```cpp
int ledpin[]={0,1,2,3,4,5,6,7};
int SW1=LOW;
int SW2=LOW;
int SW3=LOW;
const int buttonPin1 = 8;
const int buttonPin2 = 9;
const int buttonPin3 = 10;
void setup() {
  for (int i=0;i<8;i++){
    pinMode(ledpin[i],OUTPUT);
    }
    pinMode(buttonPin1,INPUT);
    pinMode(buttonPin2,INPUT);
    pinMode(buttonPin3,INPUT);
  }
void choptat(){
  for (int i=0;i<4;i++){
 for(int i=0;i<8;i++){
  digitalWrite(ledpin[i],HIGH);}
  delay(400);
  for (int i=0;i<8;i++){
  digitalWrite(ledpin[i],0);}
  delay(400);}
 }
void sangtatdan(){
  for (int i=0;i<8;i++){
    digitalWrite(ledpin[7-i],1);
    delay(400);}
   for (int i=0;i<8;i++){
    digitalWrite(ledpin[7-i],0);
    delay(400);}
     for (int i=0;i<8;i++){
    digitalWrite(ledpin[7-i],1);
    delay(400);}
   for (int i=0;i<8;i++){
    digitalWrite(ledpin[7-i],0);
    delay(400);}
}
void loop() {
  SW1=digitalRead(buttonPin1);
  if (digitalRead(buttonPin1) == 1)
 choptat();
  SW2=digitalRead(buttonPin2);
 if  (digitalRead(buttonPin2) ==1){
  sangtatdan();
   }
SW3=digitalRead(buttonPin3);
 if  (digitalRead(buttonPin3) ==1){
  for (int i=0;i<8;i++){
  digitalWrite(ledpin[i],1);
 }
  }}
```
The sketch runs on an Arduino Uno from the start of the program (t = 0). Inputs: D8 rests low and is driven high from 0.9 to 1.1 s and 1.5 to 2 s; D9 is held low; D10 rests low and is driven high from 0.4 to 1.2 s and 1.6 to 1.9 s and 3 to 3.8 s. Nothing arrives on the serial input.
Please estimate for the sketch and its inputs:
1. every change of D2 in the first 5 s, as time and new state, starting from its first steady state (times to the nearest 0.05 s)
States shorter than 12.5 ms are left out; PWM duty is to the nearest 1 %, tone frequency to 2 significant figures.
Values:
0 s low; 0.4 s high; 1.3 s low; 1.7 s high; 2.1 s low; 2.5 s high; 2.9 s low; 3.3 s high; 3.7 s low
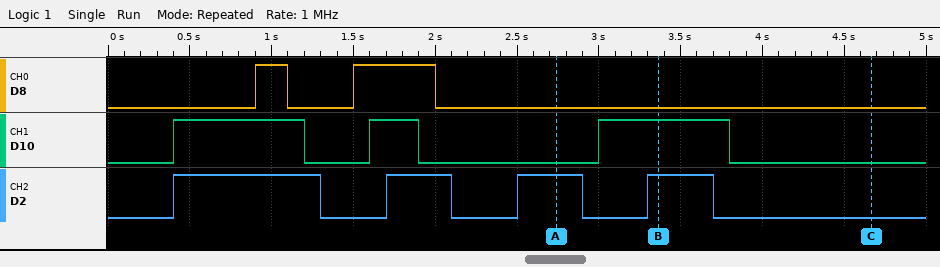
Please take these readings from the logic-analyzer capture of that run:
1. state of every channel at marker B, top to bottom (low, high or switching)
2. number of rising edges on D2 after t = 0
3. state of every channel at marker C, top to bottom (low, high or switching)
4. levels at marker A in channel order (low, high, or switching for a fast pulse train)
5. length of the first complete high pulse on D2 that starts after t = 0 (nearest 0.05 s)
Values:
D8 low, D10 high, D2 high
4
D8 low, D10 low, D2 low
D8 low, D10 low, D2 high
0.90 s
